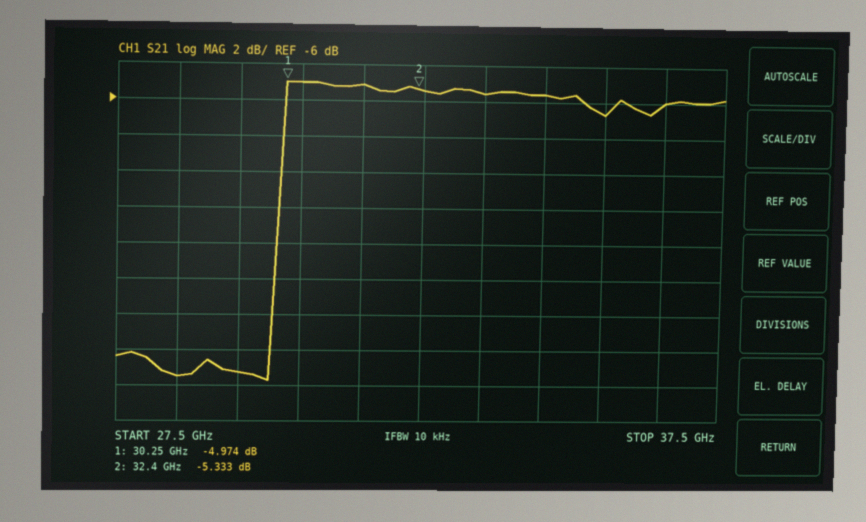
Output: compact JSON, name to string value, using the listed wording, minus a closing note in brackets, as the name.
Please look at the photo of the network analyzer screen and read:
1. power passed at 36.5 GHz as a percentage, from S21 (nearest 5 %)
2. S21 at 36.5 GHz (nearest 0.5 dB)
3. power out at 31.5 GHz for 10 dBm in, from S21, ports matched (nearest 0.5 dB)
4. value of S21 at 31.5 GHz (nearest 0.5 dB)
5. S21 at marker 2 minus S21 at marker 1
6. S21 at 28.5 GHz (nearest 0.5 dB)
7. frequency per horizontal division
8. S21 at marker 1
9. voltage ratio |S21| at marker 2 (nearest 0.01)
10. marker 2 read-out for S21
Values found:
{"power passed at 36.5 GHz as a percentage, from S21": "25 %", "S21 at 36.5 GHz": "-6.0 dB", "power out at 31.5 GHz for 10 dBm in, from S21, ports matched": "5.0 dBm", "value of S21 at 31.5 GHz": "-5.0 dB", "S21 at marker 2 minus S21 at marker 1": "-0.359 dB", "S21 at 28.5 GHz": "-21.5 dB", "frequency per horizontal division": "1 GHz", "S21 at marker 1": "-4.974 dB", "voltage ratio |S21| at marker 2": "0.54", "marker 2 read-out for S21": "-5.333 dB"}
